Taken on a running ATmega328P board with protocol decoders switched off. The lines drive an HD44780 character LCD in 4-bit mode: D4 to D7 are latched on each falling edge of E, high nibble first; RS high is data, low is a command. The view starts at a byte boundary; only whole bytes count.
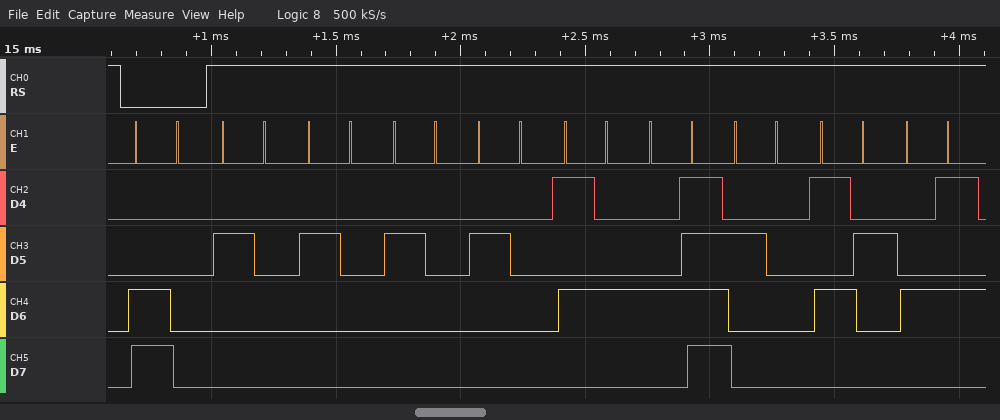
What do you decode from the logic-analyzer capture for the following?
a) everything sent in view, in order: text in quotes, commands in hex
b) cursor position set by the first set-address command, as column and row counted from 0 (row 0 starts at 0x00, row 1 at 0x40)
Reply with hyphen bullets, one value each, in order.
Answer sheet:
- 0xC0 "    TO RE"
- column 0, row 1
